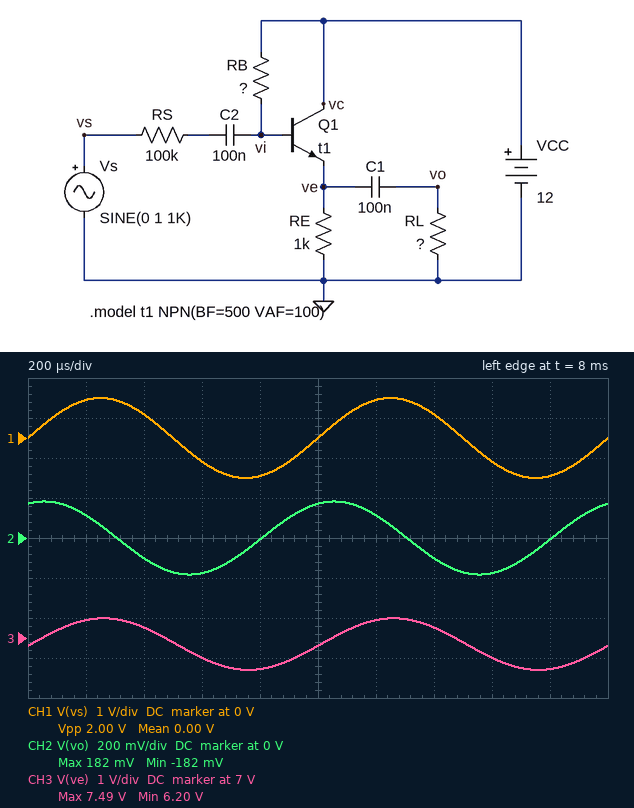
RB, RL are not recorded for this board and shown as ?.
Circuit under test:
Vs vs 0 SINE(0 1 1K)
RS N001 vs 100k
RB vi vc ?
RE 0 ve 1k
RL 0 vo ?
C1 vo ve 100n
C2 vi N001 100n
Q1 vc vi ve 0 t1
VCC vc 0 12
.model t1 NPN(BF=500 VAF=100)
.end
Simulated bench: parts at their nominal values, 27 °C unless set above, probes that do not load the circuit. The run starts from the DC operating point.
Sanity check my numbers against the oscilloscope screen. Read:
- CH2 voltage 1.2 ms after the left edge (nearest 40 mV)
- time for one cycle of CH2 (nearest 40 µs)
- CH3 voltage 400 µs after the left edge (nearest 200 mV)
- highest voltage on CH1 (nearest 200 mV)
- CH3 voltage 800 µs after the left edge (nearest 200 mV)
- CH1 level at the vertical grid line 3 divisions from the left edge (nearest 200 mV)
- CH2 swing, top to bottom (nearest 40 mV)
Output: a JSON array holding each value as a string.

["120 mV", "1.00 ms", "7.2 V", "1.0 V", "6.2 V", "-600 mV", "360 mV"]
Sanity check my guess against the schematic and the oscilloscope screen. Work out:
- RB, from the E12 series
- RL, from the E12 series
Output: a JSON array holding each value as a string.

["330 kΩ", "470 Ω"]
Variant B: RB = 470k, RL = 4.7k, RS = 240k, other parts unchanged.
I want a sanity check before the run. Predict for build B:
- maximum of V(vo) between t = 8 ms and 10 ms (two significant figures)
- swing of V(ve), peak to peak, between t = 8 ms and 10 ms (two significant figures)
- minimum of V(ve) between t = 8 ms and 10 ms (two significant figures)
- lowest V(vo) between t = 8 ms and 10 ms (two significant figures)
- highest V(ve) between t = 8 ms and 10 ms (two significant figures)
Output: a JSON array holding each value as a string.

["450 mV", "960 mV", "5.4 V", "-450 mV", "6.4 V"]
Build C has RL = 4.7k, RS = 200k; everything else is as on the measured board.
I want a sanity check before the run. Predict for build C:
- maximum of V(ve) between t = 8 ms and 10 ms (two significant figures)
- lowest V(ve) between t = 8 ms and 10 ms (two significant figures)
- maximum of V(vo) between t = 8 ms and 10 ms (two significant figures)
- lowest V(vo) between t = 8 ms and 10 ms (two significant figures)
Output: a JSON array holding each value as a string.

["7.3 V", "6.4 V", "450 mV", "-450 mV"]
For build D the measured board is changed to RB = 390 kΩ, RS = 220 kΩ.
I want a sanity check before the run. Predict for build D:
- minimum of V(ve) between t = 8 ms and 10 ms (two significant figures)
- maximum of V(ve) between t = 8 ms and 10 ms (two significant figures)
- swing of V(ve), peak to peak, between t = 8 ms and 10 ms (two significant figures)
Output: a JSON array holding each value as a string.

["5.9 V", "6.9 V", "950 mV"]
